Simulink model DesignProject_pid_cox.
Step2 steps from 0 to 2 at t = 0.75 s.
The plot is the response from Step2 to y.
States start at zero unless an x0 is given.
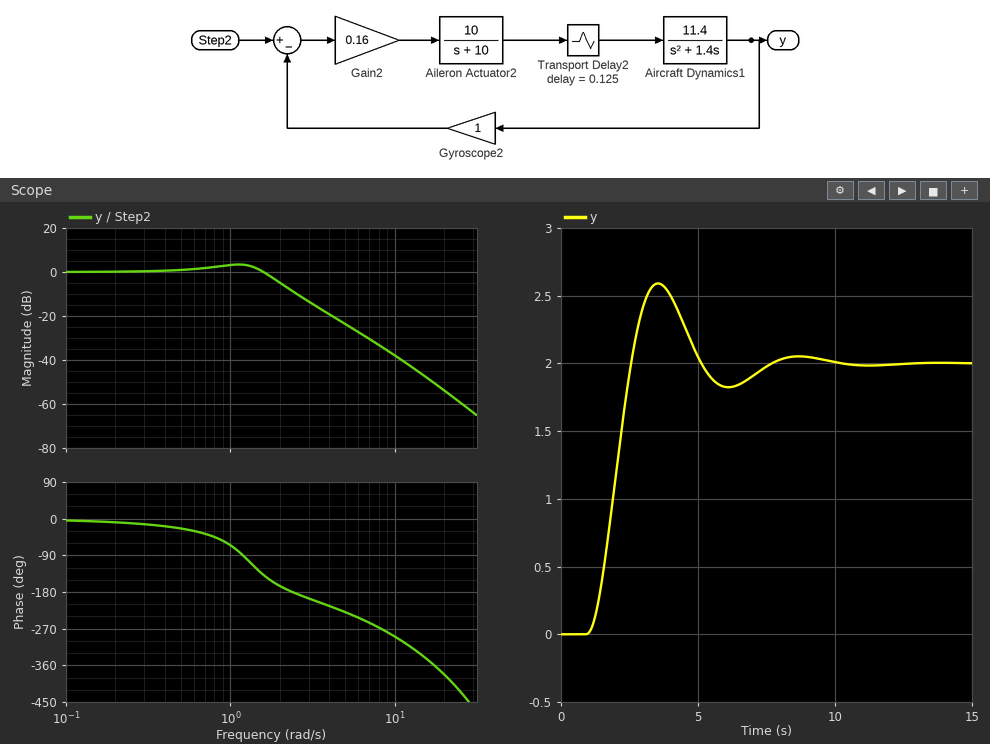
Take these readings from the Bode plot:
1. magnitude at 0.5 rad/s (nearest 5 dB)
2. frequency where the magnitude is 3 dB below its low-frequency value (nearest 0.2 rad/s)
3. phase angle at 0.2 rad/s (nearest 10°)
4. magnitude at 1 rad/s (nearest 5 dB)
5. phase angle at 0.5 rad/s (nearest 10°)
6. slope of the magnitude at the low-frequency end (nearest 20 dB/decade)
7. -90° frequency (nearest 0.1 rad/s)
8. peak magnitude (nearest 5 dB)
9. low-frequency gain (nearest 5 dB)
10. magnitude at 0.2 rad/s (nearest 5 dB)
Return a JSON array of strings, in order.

["0 dB", "1.8 rad/s", "-10°", "5 dB", "-20°", "0 dB/decade", "1.2 rad/s", "5 dB", "0 dB", "0 dB"]
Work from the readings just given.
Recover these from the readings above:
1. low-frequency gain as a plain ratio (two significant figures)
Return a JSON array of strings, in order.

["1.0"]
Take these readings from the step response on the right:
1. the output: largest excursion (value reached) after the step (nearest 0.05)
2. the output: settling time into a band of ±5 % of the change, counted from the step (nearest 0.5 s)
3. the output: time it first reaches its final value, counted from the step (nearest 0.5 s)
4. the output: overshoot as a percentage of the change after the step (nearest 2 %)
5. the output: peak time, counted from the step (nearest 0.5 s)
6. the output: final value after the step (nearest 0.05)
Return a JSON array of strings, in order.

["2.60", "6.0 s", "2.0 s", "30 %", "3.0 s", "2.00"]
